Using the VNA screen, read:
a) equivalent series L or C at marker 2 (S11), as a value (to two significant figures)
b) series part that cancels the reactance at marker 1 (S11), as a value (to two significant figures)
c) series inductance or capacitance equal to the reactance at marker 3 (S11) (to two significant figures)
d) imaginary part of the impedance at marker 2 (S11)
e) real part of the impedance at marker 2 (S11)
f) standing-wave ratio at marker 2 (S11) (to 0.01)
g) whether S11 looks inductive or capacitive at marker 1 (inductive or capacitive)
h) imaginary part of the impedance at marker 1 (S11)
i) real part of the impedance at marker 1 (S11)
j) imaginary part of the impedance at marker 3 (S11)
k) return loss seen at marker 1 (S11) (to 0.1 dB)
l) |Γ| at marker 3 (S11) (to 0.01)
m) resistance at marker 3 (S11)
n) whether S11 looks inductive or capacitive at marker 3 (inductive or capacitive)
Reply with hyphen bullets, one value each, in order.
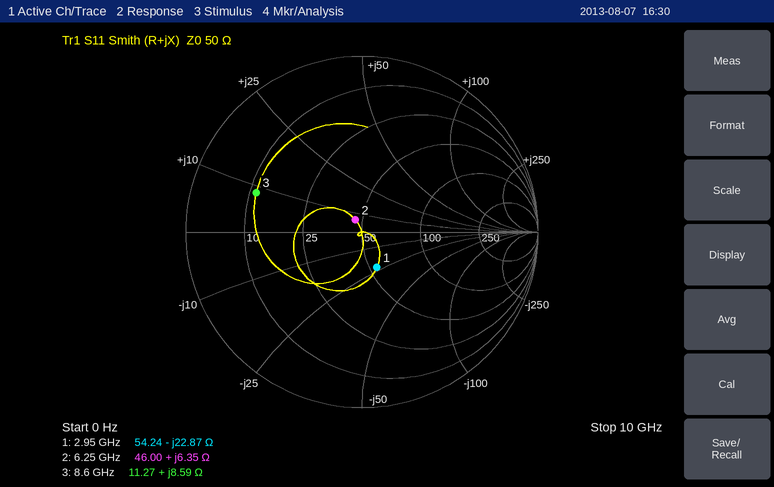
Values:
- 160 pH
- 1.2 nH
- 160 pH
- +6.35 Ω
- 46.00 Ω
- 1.17
- capacitive
- -22.87 Ω
- 54.24 Ω
- +8.59 Ω
- 13.2 dB
- 0.64
- 11.27 Ω
- inductive
